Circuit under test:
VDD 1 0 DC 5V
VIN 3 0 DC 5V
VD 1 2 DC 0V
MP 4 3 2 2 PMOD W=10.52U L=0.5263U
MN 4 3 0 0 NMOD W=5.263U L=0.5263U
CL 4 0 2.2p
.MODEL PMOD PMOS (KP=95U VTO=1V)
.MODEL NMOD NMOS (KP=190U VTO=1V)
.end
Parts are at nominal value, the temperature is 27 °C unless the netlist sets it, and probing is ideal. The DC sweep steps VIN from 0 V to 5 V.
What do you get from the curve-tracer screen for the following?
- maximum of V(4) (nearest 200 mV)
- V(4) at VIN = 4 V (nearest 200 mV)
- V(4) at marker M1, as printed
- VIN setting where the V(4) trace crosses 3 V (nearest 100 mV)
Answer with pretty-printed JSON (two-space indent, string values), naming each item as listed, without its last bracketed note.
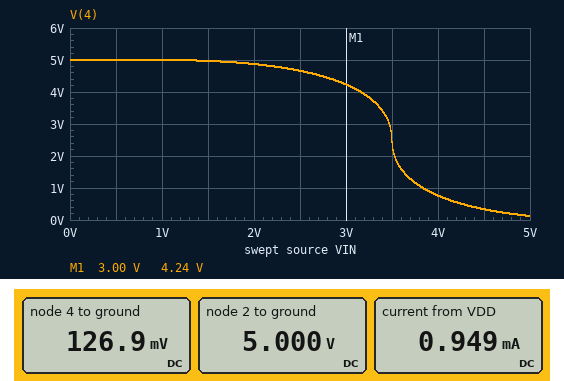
{
  "maximum of V(4)": "5.0 V",
  "V(4) at VIN = 4 V": "800 mV",
  "V(4) at marker M1, as printed": "4.24 V",
  "VIN setting where the V(4) trace crosses 3 V": "3.5 V"
}
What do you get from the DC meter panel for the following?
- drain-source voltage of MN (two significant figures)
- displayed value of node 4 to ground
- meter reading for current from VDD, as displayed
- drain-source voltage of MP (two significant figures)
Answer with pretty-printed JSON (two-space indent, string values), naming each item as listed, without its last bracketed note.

{
  "drain-source voltage of MN": "130 mV",
  "displayed value of node 4 to ground": "126.9 mV",
  "meter reading for current from VDD, as displayed": "0.949 mA",
  "drain-source voltage of MP": "-4.9 V"
}
